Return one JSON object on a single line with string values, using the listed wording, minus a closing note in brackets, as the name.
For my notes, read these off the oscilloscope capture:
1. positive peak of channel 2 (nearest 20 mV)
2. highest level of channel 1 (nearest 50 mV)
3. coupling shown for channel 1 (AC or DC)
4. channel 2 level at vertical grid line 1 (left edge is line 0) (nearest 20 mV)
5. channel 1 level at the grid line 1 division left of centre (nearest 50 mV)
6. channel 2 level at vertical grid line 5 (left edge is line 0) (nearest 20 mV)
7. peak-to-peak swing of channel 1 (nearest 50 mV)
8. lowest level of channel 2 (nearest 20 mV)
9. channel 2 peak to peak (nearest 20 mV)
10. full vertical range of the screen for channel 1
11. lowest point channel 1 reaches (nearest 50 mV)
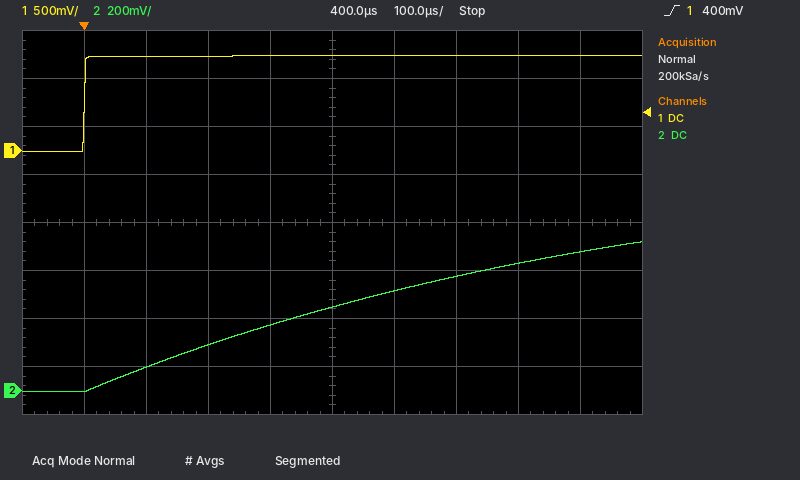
{"positive peak of channel 2": "620 mV", "highest level of channel 1": "1.00 V", "coupling shown for channel 1": "DC", "channel 2 level at vertical grid line 1 (left edge is line 0)": "0 mV", "channel 1 level at the grid line 1 division left of centre": "1.00 V", "channel 2 level at vertical grid line 5 (left edge is line 0)": "340 mV", "peak-to-peak swing of channel 1": "1.00 V", "lowest level of channel 2": "0 mV", "channel 2 peak to peak": "620 mV", "full vertical range of the screen for channel 1": "4 V", "lowest point channel 1 reaches": "0 mV"}
